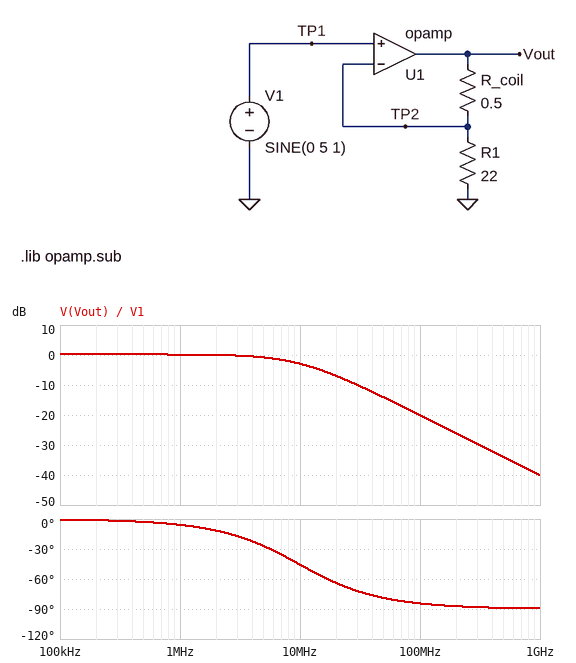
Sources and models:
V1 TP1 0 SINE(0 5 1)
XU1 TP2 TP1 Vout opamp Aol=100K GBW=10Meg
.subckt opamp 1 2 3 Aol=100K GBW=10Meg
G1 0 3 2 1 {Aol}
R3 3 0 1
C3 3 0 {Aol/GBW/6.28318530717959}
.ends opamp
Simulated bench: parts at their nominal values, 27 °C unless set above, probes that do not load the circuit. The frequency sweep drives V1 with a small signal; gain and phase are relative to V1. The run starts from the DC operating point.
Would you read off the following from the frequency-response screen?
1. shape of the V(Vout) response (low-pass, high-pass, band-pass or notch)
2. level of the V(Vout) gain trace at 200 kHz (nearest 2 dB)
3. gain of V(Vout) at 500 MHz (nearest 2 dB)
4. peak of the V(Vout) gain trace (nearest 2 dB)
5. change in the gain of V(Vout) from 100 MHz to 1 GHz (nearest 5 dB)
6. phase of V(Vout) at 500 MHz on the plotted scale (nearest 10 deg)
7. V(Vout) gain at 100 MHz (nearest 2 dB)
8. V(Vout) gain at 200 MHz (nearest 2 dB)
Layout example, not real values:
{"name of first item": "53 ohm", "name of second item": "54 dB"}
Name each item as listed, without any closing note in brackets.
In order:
{"shape of the V(Vout) response": "low-pass", "level of the V(Vout) gain trace at 200 kHz": "0 dB", "gain of V(Vout) at 500 MHz": "-34 dB", "peak of the V(Vout) gain trace": "0 dB", "change in the gain of V(Vout) from 100 MHz to 1 GHz": "-20 dB", "phase of V(Vout) at 500 MHz on the plotted scale": "-90 deg", "V(Vout) gain at 100 MHz": "-20 dB", "V(Vout) gain at 200 MHz": "-26 dB"}
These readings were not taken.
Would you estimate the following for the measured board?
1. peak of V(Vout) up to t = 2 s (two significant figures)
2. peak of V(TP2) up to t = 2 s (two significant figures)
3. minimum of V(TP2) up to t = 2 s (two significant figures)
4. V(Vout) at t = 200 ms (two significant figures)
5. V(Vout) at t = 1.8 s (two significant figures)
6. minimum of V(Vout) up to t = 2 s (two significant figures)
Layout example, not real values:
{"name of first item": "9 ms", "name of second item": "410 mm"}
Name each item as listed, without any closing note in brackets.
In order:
{"peak of V(Vout) up to t = 2 s": "5.1 V", "peak of V(TP2) up to t = 2 s": "5.0 V", "minimum of V(TP2) up to t = 2 s": "-5.0 V", "V(Vout) at t = 200 ms": "4.9 V", "V(Vout) at t = 1.8 s": "-4.9 V", "minimum of V(Vout) up to t = 2 s": "-5.1 V"}
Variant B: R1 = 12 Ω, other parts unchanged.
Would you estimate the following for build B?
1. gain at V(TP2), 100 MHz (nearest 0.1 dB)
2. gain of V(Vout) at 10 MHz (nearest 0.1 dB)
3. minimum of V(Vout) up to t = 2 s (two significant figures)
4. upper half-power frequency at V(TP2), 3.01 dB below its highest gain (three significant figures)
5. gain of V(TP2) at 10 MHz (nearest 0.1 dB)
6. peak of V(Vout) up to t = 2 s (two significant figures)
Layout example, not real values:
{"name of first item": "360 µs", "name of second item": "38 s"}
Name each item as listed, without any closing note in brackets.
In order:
{"gain at V(TP2), 100 MHz": "-20.4 dB", "gain of V(Vout) at 10 MHz": "-2.8 dB", "minimum of V(Vout) up to t = 2 s": "-5.2 V", "upper half-power frequency at V(TP2), 3.01 dB below its highest gain": "9.60 MHz", "gain of V(TP2) at 10 MHz": "-3.2 dB", "peak of V(Vout) up to t = 2 s": "5.2 V"}
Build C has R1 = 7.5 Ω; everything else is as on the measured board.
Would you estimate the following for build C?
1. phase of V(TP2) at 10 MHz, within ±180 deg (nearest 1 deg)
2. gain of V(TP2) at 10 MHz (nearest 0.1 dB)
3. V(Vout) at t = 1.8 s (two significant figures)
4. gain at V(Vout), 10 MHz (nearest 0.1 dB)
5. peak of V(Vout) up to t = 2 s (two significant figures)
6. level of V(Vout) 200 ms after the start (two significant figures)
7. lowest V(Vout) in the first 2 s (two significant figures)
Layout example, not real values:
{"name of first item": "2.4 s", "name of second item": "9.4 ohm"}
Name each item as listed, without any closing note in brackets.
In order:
{"phase of V(TP2) at 10 MHz, within ±180 deg": "-47 deg", "gain of V(TP2) at 10 MHz": "-3.3 dB", "V(Vout) at t = 1.8 s": "-5.1 V", "gain at V(Vout), 10 MHz": "-2.7 dB", "peak of V(Vout) up to t = 2 s": "5.3 V", "level of V(Vout) 200 ms after the start": "5.1 V", "lowest V(Vout) in the first 2 s": "-5.3 V"}
